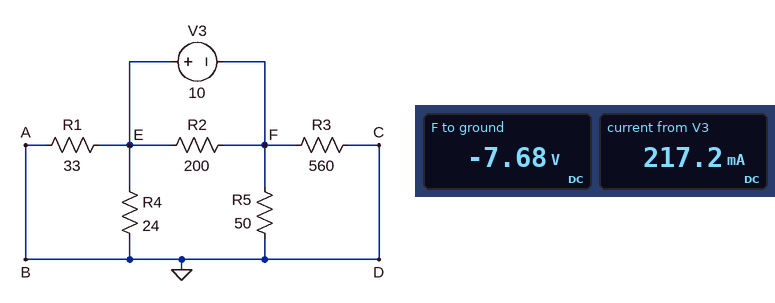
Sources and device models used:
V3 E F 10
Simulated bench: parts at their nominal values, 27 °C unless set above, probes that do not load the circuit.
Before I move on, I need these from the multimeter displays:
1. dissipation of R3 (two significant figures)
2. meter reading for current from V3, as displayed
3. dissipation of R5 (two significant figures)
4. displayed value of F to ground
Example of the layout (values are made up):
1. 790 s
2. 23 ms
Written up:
1. 110 mW
2. 217.2 mA
3. 1.2 W
4. -7.68 V
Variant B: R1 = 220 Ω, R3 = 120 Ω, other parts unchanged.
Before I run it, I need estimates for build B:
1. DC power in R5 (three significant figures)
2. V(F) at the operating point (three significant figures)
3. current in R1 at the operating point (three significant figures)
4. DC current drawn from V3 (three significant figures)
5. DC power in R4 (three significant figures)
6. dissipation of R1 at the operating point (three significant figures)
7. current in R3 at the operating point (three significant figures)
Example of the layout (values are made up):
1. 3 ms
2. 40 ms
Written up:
1. 769 mW
2. -6.20 V
3. 17.3 mA
4. 226 mA
5. 602 mW
6. 65.7 mW
7. 51.7 mA
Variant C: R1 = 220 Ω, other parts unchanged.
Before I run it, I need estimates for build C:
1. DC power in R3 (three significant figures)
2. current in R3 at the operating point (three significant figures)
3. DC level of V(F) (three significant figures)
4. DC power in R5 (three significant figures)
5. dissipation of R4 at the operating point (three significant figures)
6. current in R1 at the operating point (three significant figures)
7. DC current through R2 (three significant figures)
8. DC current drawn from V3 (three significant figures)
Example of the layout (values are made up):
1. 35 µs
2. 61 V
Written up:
1. 82.5 mW
2. 12.1 mA
3. -6.80 V
4. 924 mW
5. 428 mW
6. 14.6 mA
7. 50.0 mA
8. 198 mA
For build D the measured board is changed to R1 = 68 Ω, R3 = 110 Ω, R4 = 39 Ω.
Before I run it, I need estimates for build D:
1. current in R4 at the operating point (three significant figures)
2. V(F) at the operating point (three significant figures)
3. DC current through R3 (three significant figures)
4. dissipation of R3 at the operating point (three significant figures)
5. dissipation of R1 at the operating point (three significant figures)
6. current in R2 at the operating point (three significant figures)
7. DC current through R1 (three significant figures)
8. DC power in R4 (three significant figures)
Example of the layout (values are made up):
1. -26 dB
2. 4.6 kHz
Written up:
1. 107 mA
2. -5.81 V
3. 52.8 mA
4. 307 mW
5. 258 mW
6. 50.0 mA
7. 61.6 mA
8. 450 mW
